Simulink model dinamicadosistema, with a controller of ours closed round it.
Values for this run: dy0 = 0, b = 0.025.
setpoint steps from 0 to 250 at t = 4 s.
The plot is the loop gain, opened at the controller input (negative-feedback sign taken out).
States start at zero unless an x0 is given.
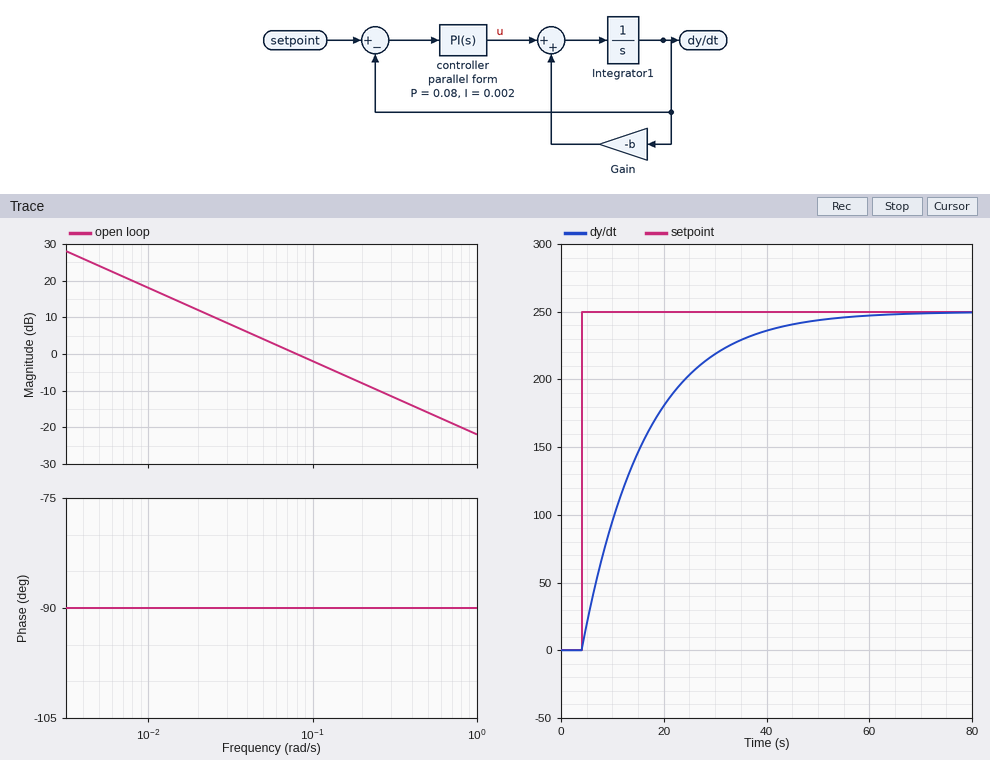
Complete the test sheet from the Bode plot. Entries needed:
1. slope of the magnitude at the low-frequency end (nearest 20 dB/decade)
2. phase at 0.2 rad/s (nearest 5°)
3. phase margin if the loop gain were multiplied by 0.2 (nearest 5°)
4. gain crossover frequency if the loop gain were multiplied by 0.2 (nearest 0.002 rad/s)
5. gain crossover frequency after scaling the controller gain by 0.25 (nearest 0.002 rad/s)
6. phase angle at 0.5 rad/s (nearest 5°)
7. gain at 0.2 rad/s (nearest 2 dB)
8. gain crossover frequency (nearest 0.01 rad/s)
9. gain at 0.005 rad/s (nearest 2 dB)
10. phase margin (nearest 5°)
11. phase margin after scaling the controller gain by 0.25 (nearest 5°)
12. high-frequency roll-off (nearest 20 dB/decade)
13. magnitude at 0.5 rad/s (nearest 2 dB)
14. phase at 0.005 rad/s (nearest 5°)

-20 dB/decade
-90°
90°
0.016 rad/s
0.020 rad/s
-90°
-8 dB
0.08 rad/s
24 dB
90°
90°
-20 dB/decade
-16 dB
-90°
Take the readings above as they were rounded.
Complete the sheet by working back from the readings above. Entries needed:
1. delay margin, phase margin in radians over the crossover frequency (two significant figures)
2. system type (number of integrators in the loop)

20 s
1
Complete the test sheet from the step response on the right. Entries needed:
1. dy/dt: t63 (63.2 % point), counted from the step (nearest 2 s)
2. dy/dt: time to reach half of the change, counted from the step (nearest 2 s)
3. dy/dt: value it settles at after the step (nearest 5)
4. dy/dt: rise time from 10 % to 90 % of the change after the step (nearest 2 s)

12 s
8 s
250
28 s
